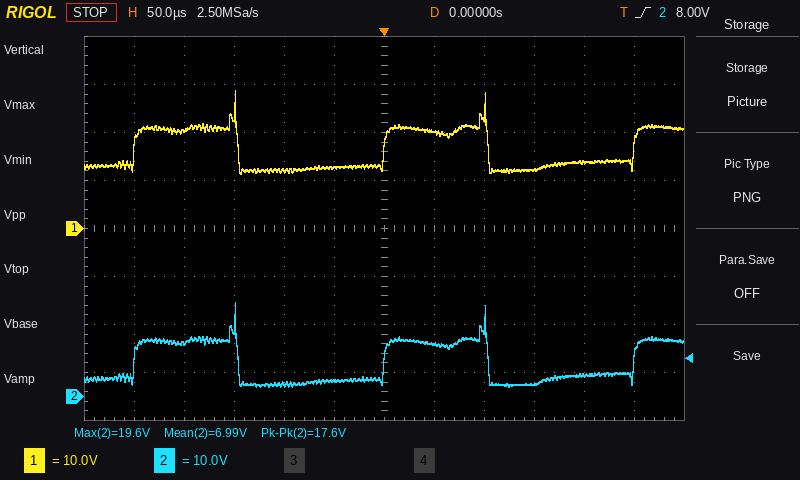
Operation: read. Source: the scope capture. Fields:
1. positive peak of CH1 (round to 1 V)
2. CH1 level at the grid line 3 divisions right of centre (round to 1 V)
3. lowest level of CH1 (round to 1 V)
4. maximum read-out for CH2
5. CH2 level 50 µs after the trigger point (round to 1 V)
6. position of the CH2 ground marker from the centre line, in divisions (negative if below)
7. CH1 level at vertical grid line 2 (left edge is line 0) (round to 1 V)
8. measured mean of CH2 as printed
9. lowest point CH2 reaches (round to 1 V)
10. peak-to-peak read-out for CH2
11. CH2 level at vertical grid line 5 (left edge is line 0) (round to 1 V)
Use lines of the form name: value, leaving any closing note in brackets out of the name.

positive peak of CH1: 29 V
CH1 level at the grid line 3 divisions right of centre: 12 V
lowest level of CH1: 11 V
maximum read-out for CH2: 19.6 V
CH2 level 50 µs after the trigger point: 11 V
position of the CH2 ground marker from the centre line, in divisions: -3.5 div
CH1 level at vertical grid line 2 (left edge is line 0): 20 V
measured mean of CH2 as printed: 6.99 V
lowest point CH2 reaches: 2 V
peak-to-peak read-out for CH2: 17.6 V
CH2 level at vertical grid line 5 (left edge is line 0): 3 V
